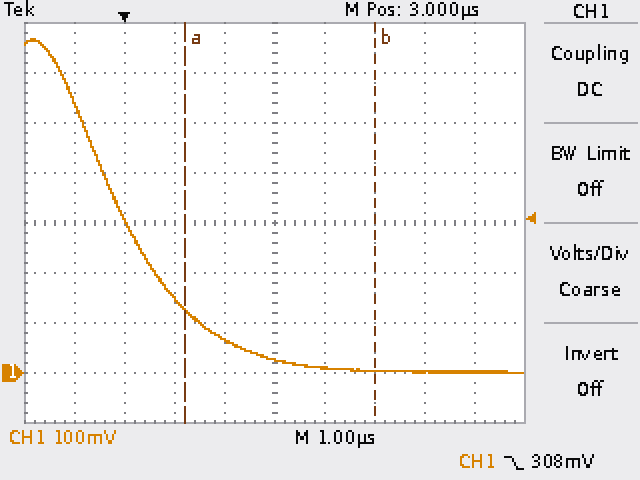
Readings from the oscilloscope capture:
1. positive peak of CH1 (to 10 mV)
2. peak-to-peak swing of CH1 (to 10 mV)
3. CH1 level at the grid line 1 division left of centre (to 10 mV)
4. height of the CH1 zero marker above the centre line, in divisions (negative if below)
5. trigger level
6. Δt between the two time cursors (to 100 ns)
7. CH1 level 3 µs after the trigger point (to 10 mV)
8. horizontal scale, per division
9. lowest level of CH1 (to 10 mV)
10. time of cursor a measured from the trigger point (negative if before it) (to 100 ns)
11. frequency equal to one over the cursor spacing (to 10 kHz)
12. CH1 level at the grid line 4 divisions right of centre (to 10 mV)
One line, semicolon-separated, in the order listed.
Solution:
670 mV; 670 mV; 70 mV; -3.0 div; 308 mV; 3.8 µs; 30 mV; 1 µs; 0 mV; +1.2 µs; 260 kHz; 0 mV
